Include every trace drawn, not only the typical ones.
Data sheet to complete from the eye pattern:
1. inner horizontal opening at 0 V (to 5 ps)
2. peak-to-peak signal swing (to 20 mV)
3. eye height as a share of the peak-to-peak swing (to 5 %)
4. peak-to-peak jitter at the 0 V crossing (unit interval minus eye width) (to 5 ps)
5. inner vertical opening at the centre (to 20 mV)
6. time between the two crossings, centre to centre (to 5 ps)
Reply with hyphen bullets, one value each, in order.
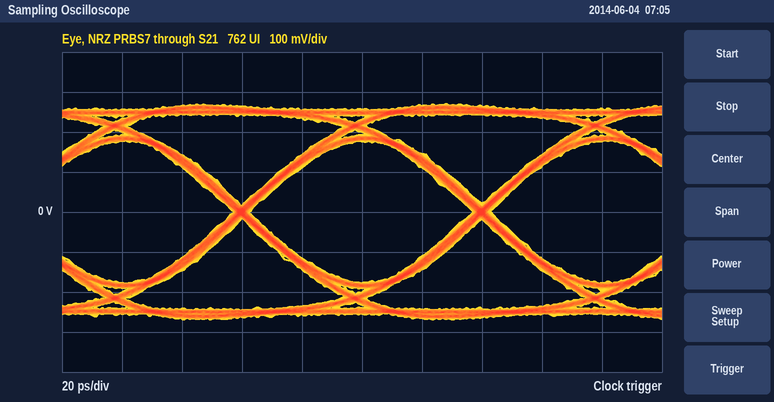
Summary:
- 75 ps
- 540 mV
- 65 %
- 5 ps
- 360 mV
- 80 ps
